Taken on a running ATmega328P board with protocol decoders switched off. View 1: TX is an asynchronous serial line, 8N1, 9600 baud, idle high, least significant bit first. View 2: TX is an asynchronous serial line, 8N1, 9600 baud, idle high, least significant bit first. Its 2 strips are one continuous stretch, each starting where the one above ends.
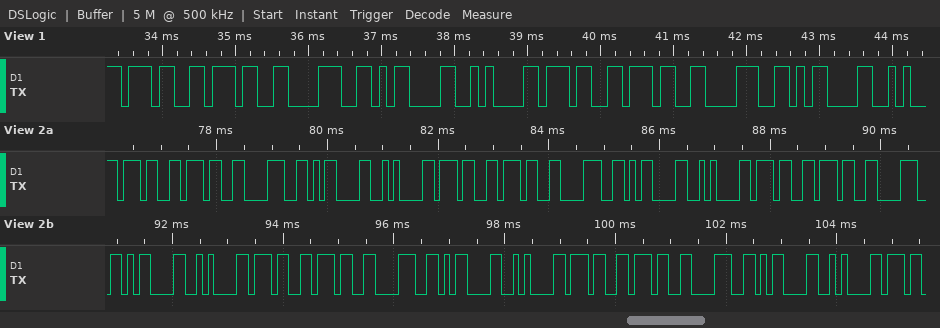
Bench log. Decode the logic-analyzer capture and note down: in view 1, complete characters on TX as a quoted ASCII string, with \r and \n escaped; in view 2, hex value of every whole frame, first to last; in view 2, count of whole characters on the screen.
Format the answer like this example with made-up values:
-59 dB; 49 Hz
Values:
"778\r\n778\r"; 0x37 0x37 0x38 0x0D 0x0A 0x37 0x37 0x38 0x0D 0x0A 0x37 0x37 0x38 0x0D 0x0A 0x37 0x37 0x38 0x0D 0x0A 0x37 0x37 0x38 0x0D 0x0A; 25
